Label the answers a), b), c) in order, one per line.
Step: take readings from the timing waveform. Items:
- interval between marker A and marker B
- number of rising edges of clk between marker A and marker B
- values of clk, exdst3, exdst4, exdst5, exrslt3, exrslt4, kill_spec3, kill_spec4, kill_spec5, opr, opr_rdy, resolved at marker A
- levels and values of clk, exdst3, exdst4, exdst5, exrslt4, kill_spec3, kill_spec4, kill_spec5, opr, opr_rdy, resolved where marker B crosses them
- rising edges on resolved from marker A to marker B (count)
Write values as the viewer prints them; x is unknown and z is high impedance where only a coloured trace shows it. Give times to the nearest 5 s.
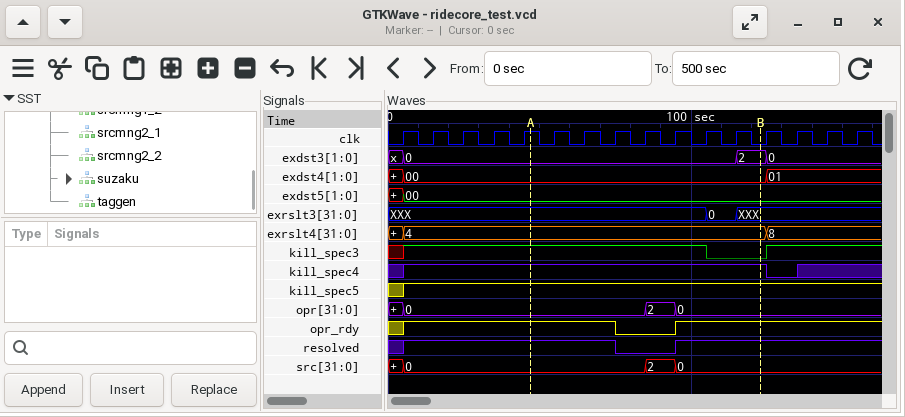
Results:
a) 75 s
b) 7
c) clk=1, exdst3=0, exdst4=00, exdst5=00, exrslt3=XXX, exrslt4=4, kill_spec3=1, kill_spec4=1, kill_spec5=1, opr=0, opr_rdy=1, resolved=1
d) clk=0, exdst3=2, exdst4=00, exdst5=00, exrslt4=4, kill_spec3=0, kill_spec4=1, kill_spec5=1, opr=0, opr_rdy=1, resolved=1
e) 1
